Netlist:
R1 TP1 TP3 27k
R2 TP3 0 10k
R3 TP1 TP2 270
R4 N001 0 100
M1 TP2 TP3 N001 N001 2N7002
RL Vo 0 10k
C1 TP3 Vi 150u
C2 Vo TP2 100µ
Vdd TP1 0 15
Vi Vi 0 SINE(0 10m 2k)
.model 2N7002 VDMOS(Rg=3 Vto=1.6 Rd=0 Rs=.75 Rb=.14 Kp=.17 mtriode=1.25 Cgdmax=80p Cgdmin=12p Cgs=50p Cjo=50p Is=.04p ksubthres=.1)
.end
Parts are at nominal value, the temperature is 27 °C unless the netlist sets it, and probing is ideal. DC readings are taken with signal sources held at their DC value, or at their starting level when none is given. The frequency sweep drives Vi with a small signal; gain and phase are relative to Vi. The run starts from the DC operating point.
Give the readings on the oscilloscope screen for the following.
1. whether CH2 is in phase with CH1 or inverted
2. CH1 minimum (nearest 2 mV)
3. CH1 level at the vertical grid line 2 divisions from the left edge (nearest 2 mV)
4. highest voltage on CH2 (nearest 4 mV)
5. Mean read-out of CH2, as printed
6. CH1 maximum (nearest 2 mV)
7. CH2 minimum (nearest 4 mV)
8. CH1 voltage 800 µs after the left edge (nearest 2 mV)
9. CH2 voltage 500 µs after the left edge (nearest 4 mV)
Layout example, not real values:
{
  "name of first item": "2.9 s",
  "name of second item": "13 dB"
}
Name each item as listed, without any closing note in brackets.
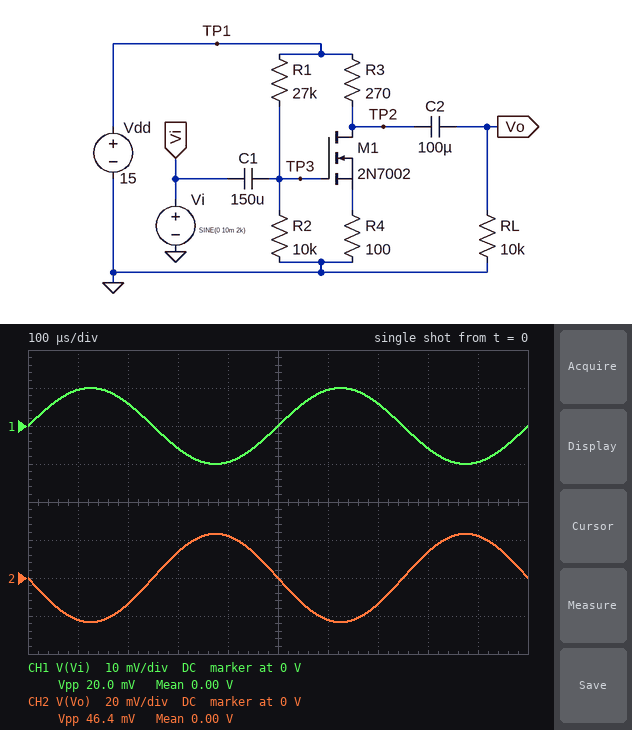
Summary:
{
  "whether CH2 is in phase with CH1 or inverted": "inverted",
  "CH1 minimum": "-10 mV",
  "CH1 level at the vertical grid line 2 divisions from the left edge": "6 mV",
  "highest voltage on CH2": "24 mV",
  "Mean read-out of CH2, as printed": "0.00 V",
  "CH1 maximum": "10 mV",
  "CH2 minimum": "-24 mV",
  "CH1 voltage 800 µs after the left edge": "-6 mV",
  "CH2 voltage 500 µs after the left edge": "0 V"
}
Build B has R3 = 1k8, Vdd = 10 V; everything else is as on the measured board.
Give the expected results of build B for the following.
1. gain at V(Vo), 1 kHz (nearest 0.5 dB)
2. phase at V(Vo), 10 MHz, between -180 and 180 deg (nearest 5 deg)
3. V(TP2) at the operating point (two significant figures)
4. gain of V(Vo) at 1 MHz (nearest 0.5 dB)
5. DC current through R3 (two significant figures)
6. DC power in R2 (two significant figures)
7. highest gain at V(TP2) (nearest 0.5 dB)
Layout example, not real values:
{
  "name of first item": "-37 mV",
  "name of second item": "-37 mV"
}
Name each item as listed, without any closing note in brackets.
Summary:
{
  "gain at V(Vo), 1 kHz": "-22.0 dB",
  "phase at V(Vo), 10 MHz, between -180 and 180 deg": "55 deg",
  "V(TP2) at the operating point": "570 mV",
  "gain of V(Vo) at 1 MHz": "-18.5 dB",
  "DC current through R3": "5.2 mA",
  "DC power in R2": "730 µW",
  "highest gain at V(TP2)": "0 dB"
}
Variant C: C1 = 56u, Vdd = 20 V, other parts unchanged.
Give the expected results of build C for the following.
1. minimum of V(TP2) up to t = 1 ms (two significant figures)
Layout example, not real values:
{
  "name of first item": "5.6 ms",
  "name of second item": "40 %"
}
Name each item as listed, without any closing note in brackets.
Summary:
{
  "minimum of V(TP2) up to t = 1 ms": "11 V"
}
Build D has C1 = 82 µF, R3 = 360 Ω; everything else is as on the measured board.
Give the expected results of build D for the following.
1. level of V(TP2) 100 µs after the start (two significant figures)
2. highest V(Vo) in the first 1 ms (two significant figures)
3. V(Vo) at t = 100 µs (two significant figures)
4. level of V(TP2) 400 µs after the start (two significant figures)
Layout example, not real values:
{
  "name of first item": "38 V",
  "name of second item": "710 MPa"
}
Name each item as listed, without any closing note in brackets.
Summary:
{
  "level of V(TP2) 100 µs after the start": "7.9 V",
  "highest V(Vo) in the first 1 ms": "31 mV",
  "V(Vo) at t = 100 µs": "-29 mV",
  "level of V(TP2) 400 µs after the start": "8.0 V"
}
